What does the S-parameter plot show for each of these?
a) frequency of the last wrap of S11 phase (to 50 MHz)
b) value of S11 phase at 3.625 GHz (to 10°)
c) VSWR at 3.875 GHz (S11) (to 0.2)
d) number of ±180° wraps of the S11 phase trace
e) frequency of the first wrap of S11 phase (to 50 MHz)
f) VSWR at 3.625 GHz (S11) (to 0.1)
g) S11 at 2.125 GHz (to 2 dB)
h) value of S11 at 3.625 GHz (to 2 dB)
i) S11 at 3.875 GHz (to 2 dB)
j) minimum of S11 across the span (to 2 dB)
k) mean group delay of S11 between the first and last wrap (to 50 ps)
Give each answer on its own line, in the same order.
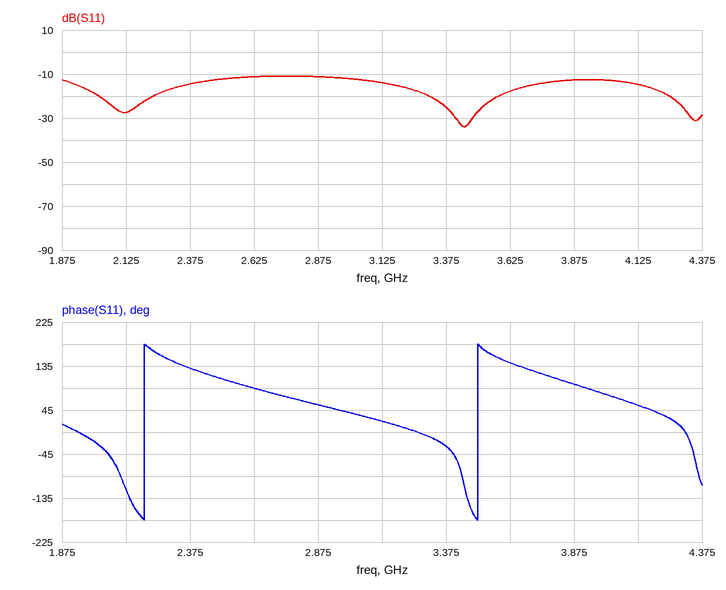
3.50 GHz
140°
1.6
2
2.20 GHz
1.3
-28 dB
-18 dB
-12 dB
-34 dB
750 ps
